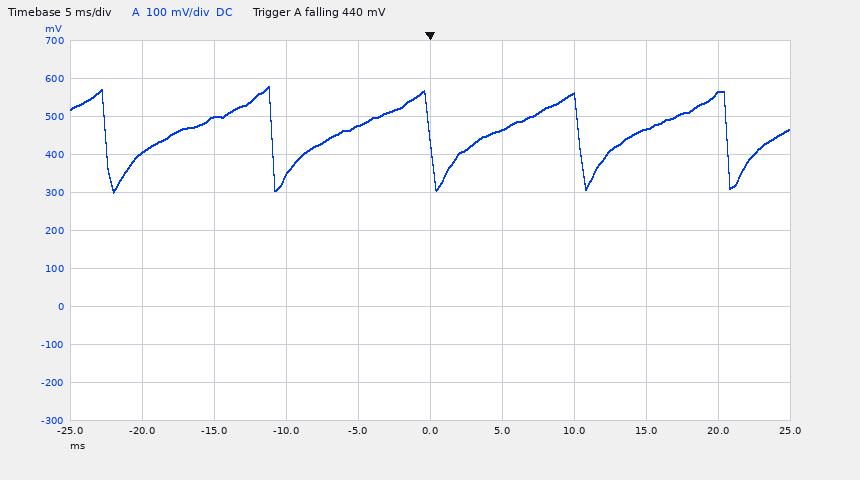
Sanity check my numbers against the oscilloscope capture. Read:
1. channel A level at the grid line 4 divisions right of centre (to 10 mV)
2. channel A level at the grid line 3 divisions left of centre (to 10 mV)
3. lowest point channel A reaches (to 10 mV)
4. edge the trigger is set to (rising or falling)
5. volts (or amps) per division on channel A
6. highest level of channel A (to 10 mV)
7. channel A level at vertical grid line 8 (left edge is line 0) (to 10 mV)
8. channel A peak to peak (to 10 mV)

560 mV
500 mV
300 mV
falling
100 mV
580 mV
470 mV
280 mV
